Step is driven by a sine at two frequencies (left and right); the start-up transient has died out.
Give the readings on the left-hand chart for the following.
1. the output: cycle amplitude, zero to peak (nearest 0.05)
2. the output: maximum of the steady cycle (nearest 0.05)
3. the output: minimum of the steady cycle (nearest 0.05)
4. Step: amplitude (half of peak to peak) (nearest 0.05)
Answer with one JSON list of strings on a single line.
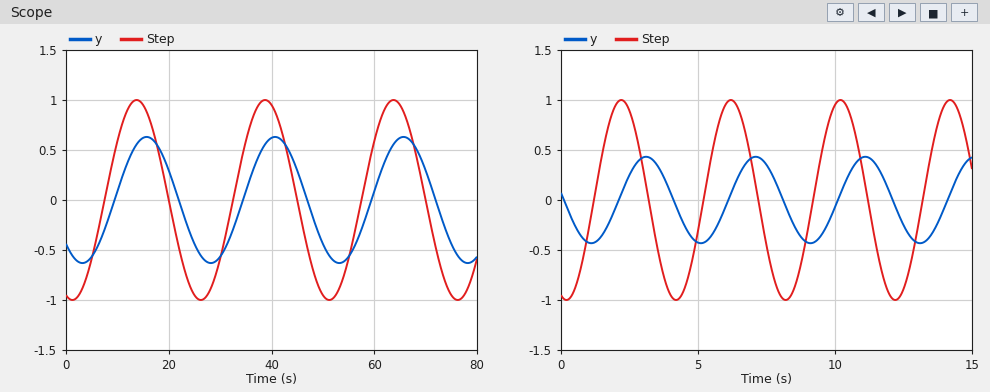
["0.65", "0.65", "-0.65", "1.00"]
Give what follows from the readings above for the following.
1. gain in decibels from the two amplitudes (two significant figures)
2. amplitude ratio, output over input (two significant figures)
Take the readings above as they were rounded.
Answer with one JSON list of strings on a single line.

["-3.7 dB", "0.65"]
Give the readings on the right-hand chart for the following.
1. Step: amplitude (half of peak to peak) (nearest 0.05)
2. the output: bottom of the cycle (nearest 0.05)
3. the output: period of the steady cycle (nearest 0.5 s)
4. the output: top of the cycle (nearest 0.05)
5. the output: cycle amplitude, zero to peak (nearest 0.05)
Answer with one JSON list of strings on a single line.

["1.00", "-0.45", "4.0 s", "0.45", "0.45"]
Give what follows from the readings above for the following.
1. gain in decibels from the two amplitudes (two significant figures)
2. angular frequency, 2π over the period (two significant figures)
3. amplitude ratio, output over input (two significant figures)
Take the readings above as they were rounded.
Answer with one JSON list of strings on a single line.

["-6.9 dB", "1.6 rad/s", "0.45"]
